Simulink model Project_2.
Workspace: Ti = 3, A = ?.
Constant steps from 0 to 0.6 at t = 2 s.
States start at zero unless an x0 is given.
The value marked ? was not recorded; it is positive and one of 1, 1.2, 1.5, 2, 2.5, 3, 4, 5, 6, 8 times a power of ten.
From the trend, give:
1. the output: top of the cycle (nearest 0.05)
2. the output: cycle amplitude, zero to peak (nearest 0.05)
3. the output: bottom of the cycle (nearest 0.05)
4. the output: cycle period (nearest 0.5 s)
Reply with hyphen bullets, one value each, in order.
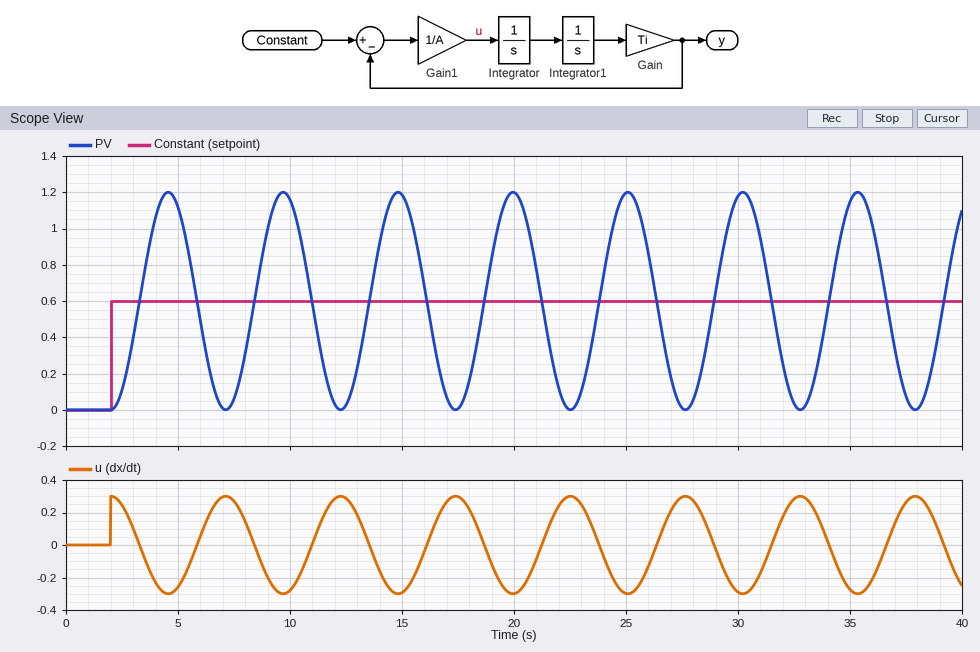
- 1.20
- 0.60
- 0.00
- 5.0 s
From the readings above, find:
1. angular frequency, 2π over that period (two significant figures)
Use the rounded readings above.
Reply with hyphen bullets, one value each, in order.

- 1.3 rad/s
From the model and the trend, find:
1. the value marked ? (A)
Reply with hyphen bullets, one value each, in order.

- 2
